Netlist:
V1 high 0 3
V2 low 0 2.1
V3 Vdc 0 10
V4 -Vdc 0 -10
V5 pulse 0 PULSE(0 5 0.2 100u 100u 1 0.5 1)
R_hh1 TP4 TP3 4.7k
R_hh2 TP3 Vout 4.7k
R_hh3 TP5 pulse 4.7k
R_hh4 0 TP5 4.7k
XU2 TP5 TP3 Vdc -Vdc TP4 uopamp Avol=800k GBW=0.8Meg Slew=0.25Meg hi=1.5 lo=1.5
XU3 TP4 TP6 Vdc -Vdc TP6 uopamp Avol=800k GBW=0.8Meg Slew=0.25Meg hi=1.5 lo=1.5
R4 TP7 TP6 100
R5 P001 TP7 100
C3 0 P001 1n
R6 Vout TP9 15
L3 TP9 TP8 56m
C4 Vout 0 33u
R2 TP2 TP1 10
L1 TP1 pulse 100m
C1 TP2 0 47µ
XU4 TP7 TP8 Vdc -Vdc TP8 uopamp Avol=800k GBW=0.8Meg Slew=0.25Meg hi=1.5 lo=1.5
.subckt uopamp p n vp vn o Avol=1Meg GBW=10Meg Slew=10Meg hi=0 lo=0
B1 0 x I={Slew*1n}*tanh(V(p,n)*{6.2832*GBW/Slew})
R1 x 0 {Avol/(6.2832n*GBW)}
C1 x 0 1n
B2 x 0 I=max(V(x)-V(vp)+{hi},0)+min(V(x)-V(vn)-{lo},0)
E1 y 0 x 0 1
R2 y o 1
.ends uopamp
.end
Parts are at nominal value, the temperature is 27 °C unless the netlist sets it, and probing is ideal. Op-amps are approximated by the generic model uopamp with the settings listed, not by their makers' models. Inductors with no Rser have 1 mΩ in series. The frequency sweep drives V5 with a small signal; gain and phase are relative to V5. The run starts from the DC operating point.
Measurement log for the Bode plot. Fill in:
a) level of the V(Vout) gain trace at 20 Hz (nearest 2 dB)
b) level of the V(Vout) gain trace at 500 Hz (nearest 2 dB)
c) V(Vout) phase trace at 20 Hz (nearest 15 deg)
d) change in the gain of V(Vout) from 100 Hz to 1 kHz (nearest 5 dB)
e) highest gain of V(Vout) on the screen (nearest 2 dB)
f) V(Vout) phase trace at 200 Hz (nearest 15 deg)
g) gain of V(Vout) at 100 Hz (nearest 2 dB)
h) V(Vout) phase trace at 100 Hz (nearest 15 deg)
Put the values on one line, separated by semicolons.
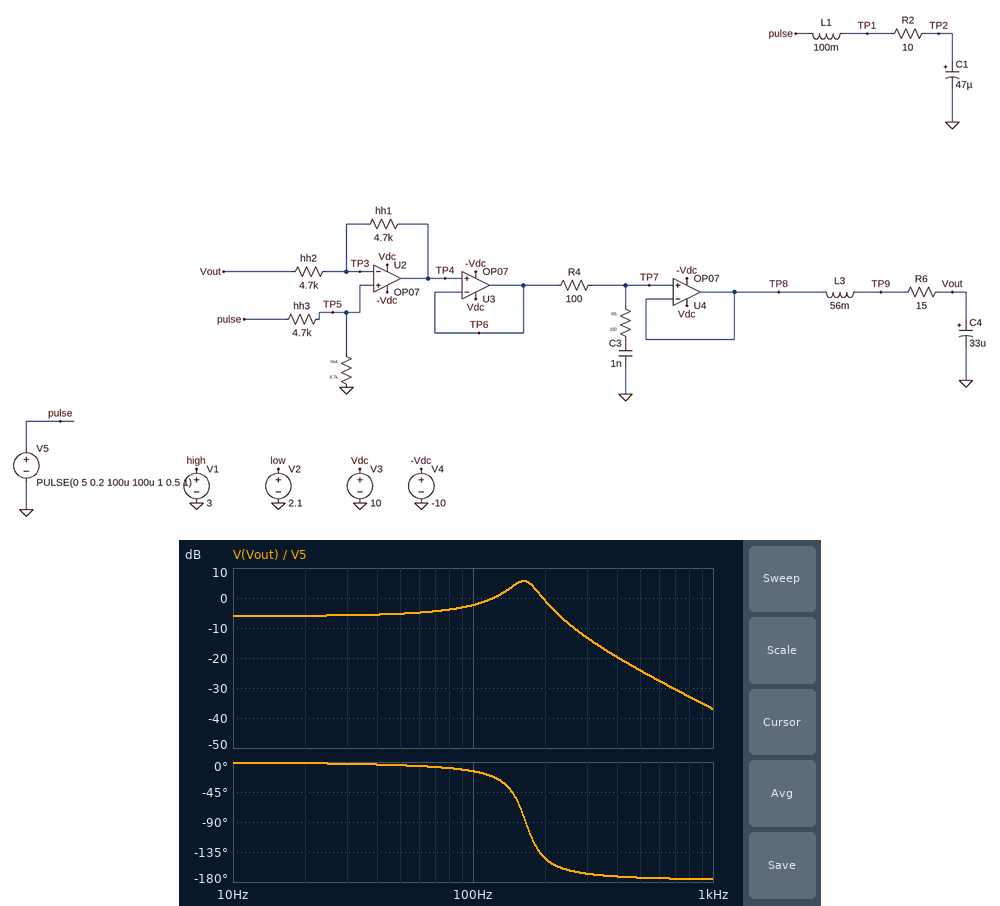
-6 dB; -24 dB; 0 deg; -35 dB; 6 dB; -150 deg; -2 dB; -15 deg
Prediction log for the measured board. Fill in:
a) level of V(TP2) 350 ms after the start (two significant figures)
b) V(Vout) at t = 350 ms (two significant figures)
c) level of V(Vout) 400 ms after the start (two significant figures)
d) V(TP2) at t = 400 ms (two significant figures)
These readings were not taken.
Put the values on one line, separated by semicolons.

5.0 V; 2.5 V; 2.5 V; 5.0 V
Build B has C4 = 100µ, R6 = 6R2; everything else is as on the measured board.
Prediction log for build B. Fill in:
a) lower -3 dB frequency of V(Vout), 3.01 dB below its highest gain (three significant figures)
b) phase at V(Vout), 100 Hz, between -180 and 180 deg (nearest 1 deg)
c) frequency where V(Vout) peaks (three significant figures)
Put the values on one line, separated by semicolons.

84.8 Hz; -118 deg; 94.3 Hz
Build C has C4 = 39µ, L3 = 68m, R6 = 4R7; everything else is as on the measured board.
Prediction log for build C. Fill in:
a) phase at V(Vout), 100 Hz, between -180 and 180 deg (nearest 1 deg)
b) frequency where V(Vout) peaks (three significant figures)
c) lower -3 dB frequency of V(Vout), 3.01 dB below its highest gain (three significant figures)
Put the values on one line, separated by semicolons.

-7 deg; 138 Hz; 132 Hz
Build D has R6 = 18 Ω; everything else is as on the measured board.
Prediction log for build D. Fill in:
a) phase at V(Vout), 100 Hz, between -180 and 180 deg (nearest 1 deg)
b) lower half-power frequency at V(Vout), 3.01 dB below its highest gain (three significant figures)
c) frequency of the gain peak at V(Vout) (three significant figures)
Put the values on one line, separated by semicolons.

-16 deg; 133 Hz; 162 Hz
